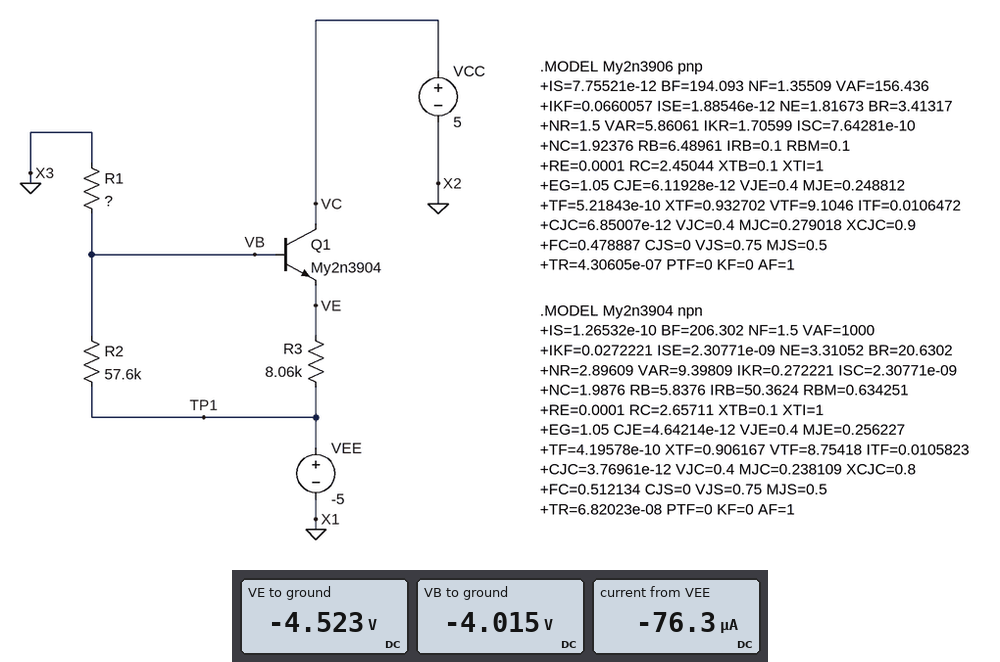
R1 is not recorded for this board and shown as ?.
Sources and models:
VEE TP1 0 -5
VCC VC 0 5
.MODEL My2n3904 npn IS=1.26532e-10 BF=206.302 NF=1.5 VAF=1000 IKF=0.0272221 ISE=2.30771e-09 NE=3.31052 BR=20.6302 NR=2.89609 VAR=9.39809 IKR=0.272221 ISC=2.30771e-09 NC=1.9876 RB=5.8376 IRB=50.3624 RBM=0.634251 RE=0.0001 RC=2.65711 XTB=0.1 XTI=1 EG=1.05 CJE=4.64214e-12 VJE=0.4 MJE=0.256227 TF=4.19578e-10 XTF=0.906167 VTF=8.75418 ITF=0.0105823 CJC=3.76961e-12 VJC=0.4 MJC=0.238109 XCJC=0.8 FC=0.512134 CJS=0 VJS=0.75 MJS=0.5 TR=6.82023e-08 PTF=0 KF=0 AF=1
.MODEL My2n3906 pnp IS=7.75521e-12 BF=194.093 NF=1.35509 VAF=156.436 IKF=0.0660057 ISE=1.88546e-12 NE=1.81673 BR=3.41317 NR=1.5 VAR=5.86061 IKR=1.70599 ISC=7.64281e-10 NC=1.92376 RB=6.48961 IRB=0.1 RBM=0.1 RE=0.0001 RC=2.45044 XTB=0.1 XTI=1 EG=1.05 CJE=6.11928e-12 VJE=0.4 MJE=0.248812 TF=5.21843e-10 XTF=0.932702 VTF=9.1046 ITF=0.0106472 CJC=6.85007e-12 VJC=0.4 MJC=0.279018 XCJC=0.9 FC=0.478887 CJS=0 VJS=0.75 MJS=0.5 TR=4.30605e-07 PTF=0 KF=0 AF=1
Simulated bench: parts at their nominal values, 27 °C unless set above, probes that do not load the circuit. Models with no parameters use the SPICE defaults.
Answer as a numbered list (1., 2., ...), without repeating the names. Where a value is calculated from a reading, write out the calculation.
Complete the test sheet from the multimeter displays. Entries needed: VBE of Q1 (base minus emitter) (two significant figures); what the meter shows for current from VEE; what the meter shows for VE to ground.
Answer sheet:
1. -4.015 V - (-4.523 V) = 510 mV
2. -76.3 µA
3. -4.523 V
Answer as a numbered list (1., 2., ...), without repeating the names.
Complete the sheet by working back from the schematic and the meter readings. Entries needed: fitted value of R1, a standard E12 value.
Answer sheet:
1. 220 kΩ
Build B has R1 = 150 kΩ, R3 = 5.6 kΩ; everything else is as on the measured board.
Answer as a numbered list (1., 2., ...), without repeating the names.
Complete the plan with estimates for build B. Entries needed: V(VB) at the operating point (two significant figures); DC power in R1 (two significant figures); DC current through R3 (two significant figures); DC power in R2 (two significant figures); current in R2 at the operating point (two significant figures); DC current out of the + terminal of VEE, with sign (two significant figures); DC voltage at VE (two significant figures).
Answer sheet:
1. -3.7 V
2. 91 µW
3. 140 µA
4. 30 µW
5. 23 µA
6. -160 µA
7. -4.2 V
